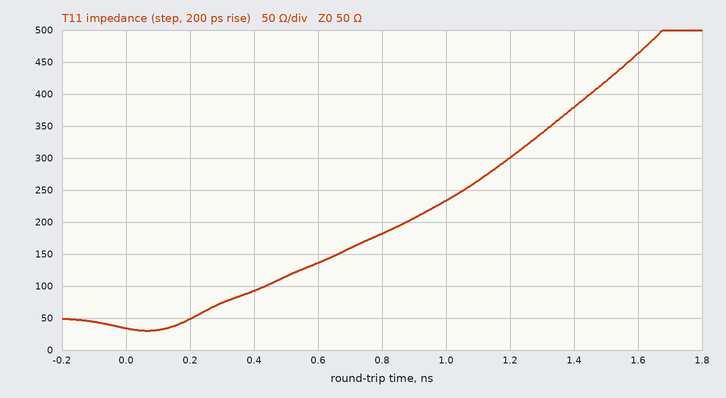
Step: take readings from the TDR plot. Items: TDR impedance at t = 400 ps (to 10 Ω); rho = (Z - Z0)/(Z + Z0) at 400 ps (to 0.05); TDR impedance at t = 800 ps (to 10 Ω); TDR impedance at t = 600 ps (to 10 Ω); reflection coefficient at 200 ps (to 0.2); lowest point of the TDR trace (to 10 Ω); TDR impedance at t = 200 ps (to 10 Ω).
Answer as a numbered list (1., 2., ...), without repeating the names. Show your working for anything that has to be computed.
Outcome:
1. 90 Ω
2. (90 − 50)/(90 + 50) ≈ +0.286, so +0.30 to the nearest 0.05
3. 180 Ω
4. 140 Ω
5. (50 − 50)/(50 + 50) ≈ 0.0
6. 30 Ω
7. 50 Ω
